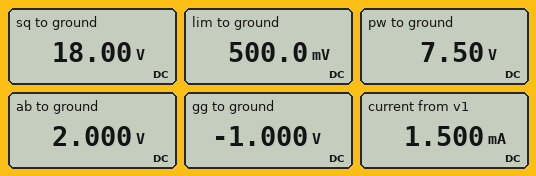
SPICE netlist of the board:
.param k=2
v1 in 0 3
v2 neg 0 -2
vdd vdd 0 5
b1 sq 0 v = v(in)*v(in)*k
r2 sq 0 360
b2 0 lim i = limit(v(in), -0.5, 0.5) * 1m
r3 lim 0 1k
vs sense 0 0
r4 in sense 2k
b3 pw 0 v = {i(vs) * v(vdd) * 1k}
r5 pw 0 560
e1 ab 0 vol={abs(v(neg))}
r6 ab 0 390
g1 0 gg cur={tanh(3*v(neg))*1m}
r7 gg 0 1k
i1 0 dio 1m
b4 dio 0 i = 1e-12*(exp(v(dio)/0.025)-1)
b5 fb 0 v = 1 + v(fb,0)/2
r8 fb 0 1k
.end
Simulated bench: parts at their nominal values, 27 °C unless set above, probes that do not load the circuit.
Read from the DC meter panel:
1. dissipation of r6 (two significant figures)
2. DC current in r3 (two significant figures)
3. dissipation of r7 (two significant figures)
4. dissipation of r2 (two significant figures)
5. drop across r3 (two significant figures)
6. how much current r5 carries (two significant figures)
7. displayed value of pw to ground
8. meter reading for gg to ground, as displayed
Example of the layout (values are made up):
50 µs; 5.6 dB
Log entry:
10 mW; 500 µA; 1.0 mW; 900 mW; 500 mV; 13 mA; 7.50 V; -1.000 V
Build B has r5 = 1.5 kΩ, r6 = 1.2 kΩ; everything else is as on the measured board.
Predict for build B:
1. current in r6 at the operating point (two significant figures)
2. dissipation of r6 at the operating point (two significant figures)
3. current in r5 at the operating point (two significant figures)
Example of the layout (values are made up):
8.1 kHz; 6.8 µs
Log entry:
1.7 mA; 3.3 mW; 5.0 mA
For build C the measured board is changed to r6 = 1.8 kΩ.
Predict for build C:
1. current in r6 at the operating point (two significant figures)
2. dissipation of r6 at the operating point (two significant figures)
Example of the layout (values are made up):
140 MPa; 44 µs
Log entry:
1.1 mA; 2.2 mW
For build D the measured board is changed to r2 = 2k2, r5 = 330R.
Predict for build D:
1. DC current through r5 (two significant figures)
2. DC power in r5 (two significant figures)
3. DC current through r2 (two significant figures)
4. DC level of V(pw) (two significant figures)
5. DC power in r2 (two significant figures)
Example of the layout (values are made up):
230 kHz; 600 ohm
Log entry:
23 mA; 170 mW; 8.2 mA; 7.5 V; 150 mW
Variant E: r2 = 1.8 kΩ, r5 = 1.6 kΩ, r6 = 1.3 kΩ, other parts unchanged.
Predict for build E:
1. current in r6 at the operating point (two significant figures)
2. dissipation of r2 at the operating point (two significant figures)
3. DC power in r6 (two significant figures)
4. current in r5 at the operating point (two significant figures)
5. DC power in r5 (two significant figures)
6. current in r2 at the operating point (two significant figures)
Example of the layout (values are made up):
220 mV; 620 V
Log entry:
1.5 mA; 180 mW; 3.1 mW; 4.7 mA; 35 mW; 10 mA
